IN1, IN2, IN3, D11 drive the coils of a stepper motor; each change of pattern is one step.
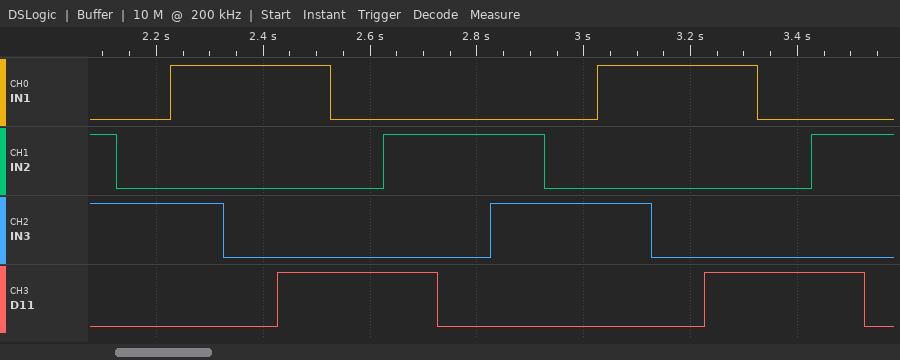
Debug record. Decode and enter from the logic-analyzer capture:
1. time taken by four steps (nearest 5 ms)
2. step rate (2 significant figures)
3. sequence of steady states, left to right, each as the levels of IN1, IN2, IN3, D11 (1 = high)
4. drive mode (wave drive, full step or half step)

400 ms
10.0 steps/s
0110 0010 1010 1000 1001 0001 0101 0100 0110 0010 1010 1000 1001 0001 0101 0100
half step
